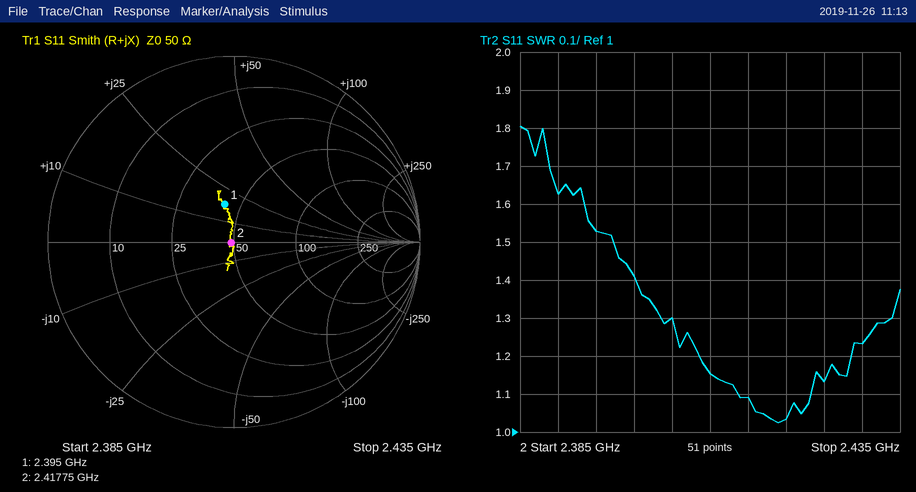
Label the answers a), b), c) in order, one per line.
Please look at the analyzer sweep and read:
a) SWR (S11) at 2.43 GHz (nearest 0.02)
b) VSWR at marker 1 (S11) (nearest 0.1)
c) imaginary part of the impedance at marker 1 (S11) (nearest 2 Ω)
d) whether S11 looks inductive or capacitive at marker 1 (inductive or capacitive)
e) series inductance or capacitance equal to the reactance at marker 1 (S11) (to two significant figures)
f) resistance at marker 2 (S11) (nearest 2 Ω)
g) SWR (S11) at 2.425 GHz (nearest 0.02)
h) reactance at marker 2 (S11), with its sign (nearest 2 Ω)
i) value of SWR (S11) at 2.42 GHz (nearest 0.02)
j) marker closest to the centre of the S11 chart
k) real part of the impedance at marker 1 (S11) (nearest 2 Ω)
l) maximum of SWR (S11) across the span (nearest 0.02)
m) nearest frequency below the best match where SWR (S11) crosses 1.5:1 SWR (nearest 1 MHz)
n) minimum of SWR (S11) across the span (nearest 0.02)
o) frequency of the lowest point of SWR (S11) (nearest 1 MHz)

a) 1.24
b) 1.5
c) +18 Ω
d) inductive
e) 1.2 nH
f) 48 Ω
g) 1.14
h) 0 Ω
i) 1.04
j) marker 2
k) 42 Ω
l) 1.80
m) 2.397 GHz
n) 1.02
o) 2.419 GHz
